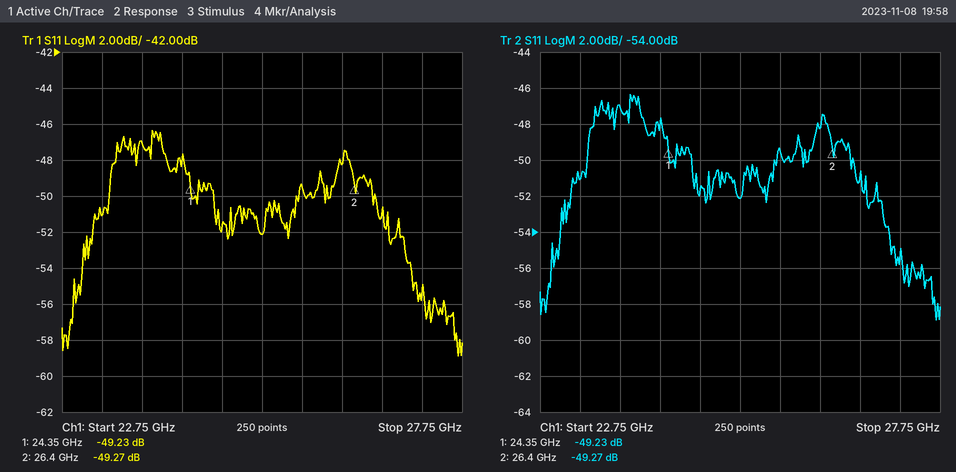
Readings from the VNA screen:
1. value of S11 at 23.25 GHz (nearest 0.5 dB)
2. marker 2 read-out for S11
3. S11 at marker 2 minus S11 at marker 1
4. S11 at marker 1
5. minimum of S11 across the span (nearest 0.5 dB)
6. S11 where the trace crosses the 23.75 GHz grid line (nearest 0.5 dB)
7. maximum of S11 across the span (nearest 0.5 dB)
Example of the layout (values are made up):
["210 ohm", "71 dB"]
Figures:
["-51.0 dB", "-49.27 dB", "-0.04 dB", "-49.23 dB", "-59.0 dB", "-47.0 dB", "-46.5 dB"]
